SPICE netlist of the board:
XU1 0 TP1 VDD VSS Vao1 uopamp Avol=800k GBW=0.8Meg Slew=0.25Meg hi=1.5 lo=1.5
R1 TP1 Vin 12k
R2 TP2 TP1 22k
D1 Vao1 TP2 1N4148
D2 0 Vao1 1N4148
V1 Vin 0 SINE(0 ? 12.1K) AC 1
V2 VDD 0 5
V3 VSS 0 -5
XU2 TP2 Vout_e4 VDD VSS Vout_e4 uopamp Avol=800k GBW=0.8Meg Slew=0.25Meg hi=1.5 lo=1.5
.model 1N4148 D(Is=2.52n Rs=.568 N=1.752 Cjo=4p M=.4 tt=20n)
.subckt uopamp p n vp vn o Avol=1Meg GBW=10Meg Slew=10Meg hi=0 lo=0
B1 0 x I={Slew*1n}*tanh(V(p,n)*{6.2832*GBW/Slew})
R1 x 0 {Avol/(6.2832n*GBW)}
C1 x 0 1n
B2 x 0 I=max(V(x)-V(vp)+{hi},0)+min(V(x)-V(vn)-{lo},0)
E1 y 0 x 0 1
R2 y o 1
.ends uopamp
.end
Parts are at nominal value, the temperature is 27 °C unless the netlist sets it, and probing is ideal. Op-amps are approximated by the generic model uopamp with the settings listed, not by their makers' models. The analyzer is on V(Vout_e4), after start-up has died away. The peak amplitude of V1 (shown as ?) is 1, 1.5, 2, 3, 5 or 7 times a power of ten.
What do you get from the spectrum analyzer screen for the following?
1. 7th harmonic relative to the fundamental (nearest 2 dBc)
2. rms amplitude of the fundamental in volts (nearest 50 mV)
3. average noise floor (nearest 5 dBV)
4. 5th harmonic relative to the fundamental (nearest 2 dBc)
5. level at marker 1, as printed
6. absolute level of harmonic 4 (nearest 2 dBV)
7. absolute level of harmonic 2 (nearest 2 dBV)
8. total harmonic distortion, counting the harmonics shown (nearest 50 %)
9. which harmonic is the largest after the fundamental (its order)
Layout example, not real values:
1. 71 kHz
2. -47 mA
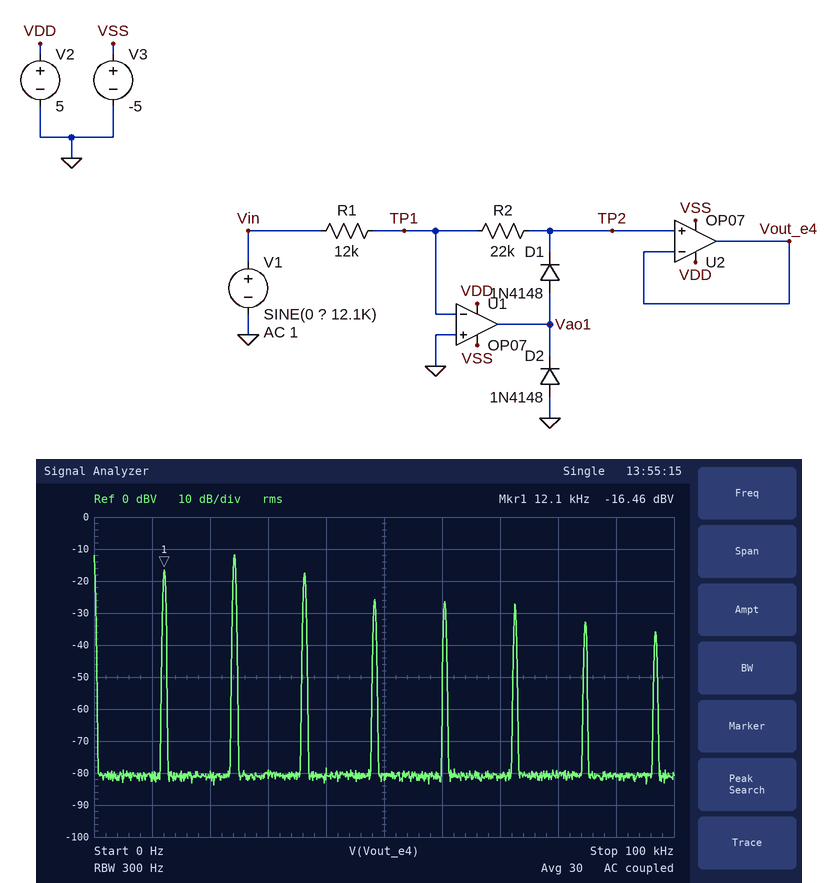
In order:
1. -16 dBc
2. 150 mV
3. -80 dBV
4. -10 dBc
5. -16.46 dBV
6. -26 dBV
7. -12 dBV
8. 200 %
9. 2
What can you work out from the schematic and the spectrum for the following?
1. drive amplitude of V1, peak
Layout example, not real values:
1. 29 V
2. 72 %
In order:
1. 500 mV
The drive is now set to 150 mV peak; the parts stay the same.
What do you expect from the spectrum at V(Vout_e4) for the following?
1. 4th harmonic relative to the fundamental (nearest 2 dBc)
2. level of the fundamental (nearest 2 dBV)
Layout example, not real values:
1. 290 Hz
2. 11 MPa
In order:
1. -8 dBc
2. -26 dBV
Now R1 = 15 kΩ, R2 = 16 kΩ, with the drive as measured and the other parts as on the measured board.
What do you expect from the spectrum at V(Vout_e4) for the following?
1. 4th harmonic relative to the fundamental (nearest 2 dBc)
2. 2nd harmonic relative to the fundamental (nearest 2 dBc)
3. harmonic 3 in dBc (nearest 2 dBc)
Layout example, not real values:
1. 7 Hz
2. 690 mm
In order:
1. -12 dBc
2. 2 dBc
3. -4 dBc
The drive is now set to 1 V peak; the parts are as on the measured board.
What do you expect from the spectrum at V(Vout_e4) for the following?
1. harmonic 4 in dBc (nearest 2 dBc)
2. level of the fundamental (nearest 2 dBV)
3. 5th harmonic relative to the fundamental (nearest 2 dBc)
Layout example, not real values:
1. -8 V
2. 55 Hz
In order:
1. -12 dBc
2. -10 dBV
3. -16 dBc
